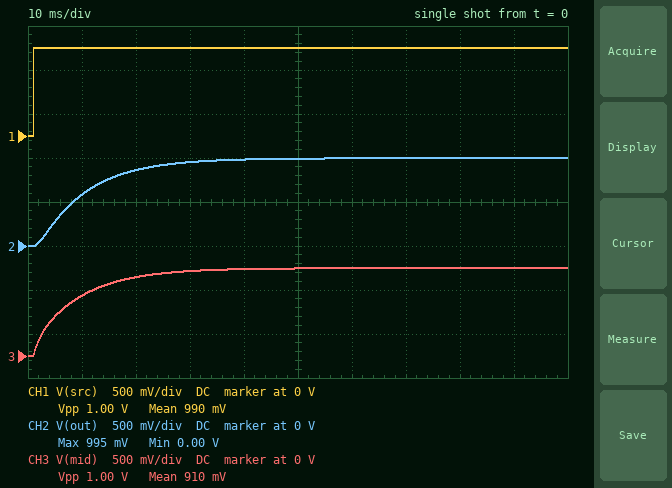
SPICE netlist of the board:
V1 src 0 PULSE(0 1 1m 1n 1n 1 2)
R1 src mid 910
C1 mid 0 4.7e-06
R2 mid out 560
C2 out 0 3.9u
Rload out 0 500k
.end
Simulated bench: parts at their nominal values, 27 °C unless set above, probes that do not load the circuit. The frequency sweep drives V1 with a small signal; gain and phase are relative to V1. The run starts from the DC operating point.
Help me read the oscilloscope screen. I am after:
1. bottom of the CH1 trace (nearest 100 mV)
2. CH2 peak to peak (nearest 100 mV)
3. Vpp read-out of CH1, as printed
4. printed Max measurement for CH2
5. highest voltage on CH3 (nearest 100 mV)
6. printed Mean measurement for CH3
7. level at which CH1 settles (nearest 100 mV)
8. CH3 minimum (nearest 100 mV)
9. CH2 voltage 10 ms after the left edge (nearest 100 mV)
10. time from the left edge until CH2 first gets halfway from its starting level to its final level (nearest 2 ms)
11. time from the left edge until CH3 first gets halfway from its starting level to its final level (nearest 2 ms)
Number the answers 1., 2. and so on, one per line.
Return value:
1. 0 V
2. 1.0 V
3. 1.00 V
4. 995 mV
5. 1.0 V
6. 910 mV
7. 1.0 V
8. 0 V
9. 600 mV
10. 8 ms
11. 6 ms
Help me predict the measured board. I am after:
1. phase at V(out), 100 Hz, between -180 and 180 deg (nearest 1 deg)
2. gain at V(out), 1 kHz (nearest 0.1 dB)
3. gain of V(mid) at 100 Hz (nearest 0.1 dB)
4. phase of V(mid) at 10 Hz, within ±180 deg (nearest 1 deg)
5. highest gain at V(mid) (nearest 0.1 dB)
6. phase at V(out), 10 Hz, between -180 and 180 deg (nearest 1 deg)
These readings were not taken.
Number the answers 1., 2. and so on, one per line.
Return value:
1. -113 deg
2. -51.4 dB
3. -12.1 dB
4. -25 deg
5. 0 dB
6. -33 deg
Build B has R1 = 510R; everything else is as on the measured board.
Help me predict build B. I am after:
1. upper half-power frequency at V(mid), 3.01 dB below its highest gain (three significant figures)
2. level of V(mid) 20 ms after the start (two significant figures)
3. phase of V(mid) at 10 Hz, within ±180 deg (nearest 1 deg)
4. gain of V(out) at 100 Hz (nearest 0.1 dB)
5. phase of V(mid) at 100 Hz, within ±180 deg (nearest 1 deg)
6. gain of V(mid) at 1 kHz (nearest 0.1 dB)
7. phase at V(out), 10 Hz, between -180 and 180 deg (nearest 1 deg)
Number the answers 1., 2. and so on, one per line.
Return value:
1. 32.4 Hz
2. 970 mV
3. -15 deg
4. -12.6 dB
5. -51 deg
6. -23.7 dB
7. -23 deg
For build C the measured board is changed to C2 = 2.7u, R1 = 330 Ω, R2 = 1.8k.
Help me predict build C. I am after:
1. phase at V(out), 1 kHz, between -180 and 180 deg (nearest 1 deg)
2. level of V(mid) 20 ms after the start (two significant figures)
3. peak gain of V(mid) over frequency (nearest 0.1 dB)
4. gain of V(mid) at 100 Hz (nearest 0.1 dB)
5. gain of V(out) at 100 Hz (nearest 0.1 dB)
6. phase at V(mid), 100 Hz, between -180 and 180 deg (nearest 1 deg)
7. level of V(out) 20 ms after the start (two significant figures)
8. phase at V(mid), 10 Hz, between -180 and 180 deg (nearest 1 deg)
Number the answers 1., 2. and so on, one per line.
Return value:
1. -171 deg
2. 990 mV
3. 0 dB
4. -3.8 dB
5. -14.0 dB
6. -41 deg
7. 940 mV
8. -8 deg
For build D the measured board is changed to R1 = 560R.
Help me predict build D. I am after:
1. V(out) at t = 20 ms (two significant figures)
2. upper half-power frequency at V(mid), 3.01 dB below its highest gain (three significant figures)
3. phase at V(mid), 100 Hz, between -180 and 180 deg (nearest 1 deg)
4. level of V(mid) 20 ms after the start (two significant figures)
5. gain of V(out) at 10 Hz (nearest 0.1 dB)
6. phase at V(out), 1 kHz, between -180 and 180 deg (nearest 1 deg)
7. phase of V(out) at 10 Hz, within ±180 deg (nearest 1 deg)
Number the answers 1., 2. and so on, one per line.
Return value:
1. 950 mV
2. 29.6 Hz
3. -52 deg
4. 970 mV
5. -0.6 dB
6. -169 deg
7. -24 deg
